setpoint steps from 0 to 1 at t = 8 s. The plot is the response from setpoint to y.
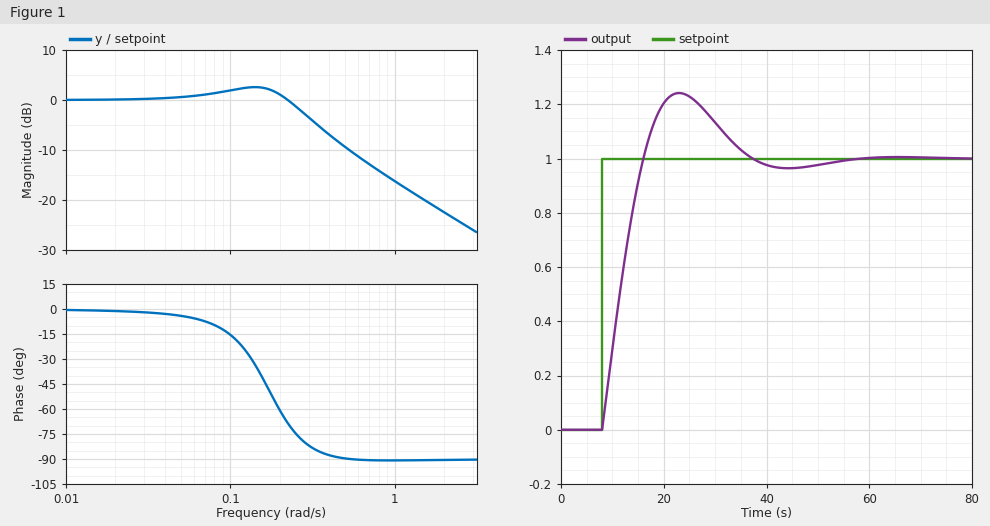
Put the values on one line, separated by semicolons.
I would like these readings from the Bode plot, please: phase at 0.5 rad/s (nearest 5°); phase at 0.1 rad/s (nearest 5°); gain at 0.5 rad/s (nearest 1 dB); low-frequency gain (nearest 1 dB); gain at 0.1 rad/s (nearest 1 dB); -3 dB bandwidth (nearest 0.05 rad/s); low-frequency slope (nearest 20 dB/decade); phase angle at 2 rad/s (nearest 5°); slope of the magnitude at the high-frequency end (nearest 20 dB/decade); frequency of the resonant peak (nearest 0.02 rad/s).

-90°; -15°; -9 dB; 0 dB; 2 dB; 0.30 rad/s; 0 dB/decade; -90°; -20 dB/decade; 0.14 rad/s
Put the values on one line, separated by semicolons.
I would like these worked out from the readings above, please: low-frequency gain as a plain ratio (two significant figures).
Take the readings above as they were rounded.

1.0
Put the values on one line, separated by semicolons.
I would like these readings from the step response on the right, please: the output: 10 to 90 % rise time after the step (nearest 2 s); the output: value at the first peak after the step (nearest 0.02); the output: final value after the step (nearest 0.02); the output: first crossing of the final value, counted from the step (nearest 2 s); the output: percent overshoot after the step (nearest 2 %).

6 s; 1.24; 1.00; 8 s; 24 %
